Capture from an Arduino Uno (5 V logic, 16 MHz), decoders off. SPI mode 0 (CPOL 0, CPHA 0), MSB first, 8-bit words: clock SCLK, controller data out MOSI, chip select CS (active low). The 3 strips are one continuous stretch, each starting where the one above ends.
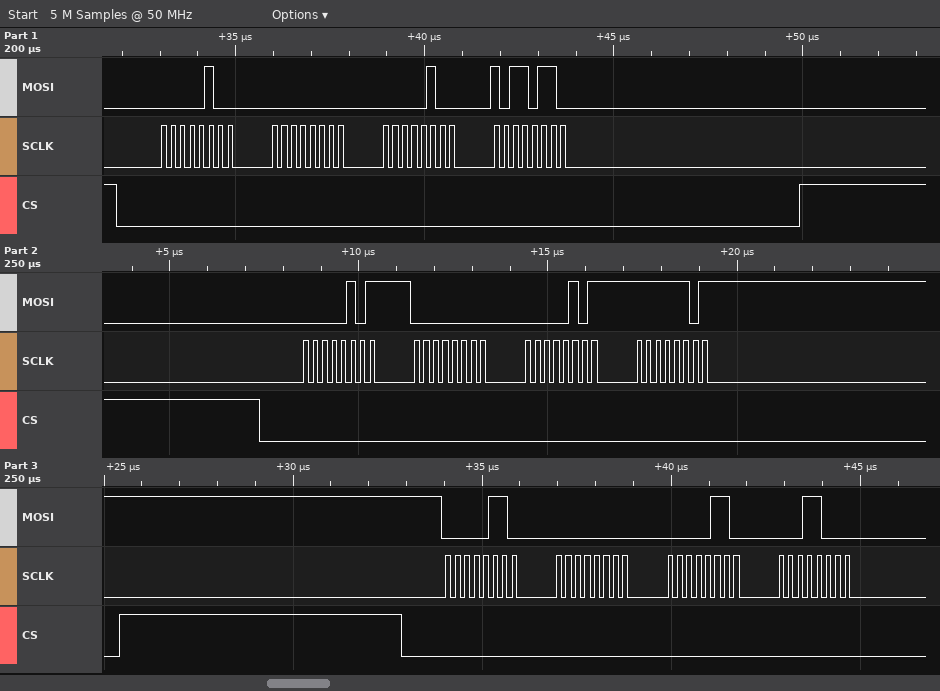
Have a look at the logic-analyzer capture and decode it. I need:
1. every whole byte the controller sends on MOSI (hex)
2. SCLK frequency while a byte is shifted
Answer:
0x04 0x00 0x04 0xB6 0x05 0x00 0x05 0xFD 0x06 0x00 0x06 0x18
4 MHz
